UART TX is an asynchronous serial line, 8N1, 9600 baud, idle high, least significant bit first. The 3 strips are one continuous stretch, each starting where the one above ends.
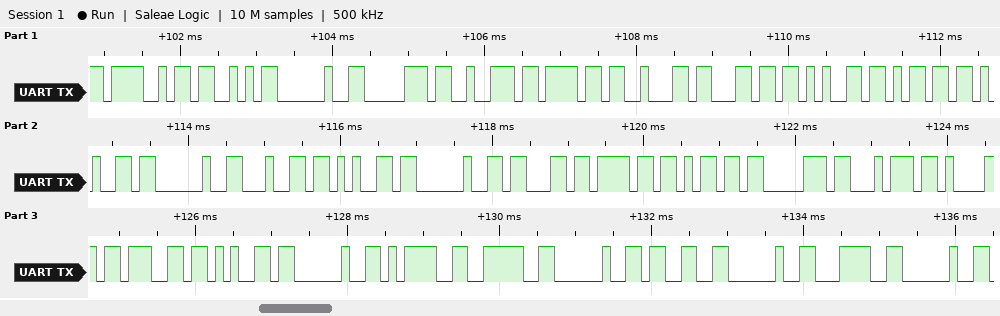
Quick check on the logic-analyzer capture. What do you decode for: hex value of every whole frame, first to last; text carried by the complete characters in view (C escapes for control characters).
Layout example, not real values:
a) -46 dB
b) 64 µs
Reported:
a) 4F 53 20 70 72 6F 62 6C 65 6D 65 20 64 65 20 63 6F 6D 70 74 61 67 65 20 3D 3E 20 33 20 3C 20
b) "OS probleme de comptage => 3 < "
